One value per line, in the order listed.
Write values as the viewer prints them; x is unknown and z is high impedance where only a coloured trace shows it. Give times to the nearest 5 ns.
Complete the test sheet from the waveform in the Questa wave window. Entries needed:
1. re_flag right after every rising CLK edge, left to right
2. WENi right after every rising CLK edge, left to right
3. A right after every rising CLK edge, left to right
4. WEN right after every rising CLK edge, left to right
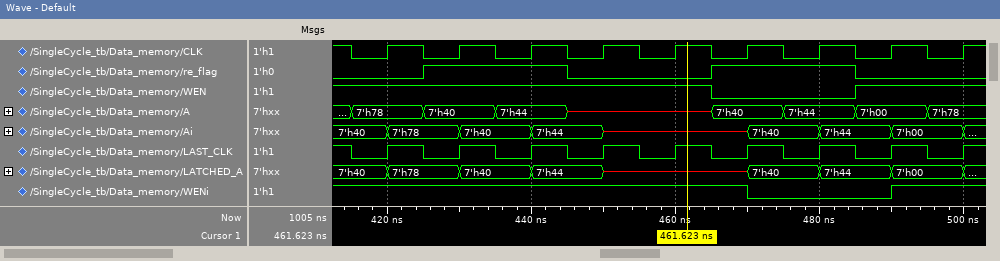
0 1 1 0 0 1 1 0 0
1 1 1 1 1 0 0 1 1
7'h78, 7'h40, 7'h44, x, x, 7'h40, 7'h44, 7'h00, 7'h78
1 1 1 1 1 0 0 1 1
